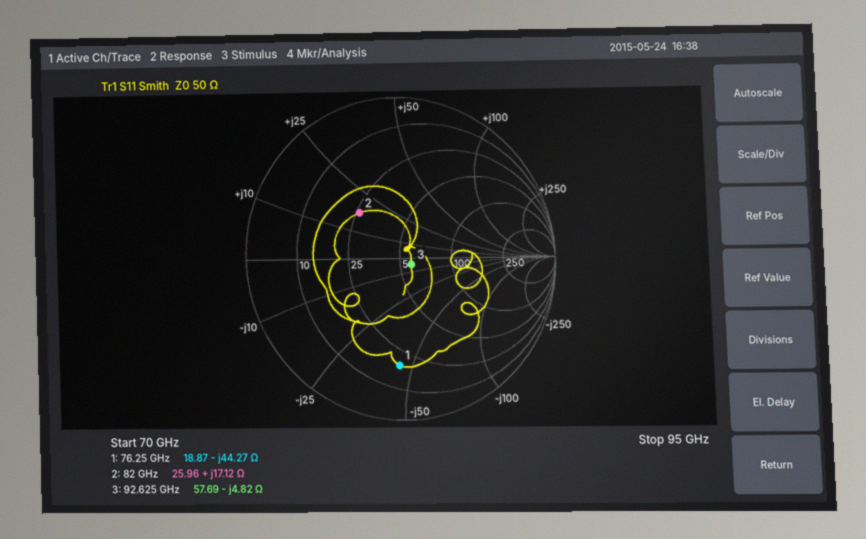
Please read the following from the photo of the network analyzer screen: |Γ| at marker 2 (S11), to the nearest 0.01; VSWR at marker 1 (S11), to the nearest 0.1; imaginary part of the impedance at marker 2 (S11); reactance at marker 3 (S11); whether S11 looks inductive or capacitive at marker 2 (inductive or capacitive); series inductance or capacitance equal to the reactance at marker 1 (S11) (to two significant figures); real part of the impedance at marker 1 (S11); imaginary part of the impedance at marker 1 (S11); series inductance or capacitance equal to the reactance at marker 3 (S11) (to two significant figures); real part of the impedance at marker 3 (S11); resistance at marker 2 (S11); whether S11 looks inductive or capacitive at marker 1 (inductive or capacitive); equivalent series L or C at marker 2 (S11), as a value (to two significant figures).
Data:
0.38
4.9
+17.12 Ω
-4.82 Ω
inductive
47 fF
18.87 Ω
-44.27 Ω
360 fF
57.69 Ω
25.96 Ω
capacitive
33 pH
